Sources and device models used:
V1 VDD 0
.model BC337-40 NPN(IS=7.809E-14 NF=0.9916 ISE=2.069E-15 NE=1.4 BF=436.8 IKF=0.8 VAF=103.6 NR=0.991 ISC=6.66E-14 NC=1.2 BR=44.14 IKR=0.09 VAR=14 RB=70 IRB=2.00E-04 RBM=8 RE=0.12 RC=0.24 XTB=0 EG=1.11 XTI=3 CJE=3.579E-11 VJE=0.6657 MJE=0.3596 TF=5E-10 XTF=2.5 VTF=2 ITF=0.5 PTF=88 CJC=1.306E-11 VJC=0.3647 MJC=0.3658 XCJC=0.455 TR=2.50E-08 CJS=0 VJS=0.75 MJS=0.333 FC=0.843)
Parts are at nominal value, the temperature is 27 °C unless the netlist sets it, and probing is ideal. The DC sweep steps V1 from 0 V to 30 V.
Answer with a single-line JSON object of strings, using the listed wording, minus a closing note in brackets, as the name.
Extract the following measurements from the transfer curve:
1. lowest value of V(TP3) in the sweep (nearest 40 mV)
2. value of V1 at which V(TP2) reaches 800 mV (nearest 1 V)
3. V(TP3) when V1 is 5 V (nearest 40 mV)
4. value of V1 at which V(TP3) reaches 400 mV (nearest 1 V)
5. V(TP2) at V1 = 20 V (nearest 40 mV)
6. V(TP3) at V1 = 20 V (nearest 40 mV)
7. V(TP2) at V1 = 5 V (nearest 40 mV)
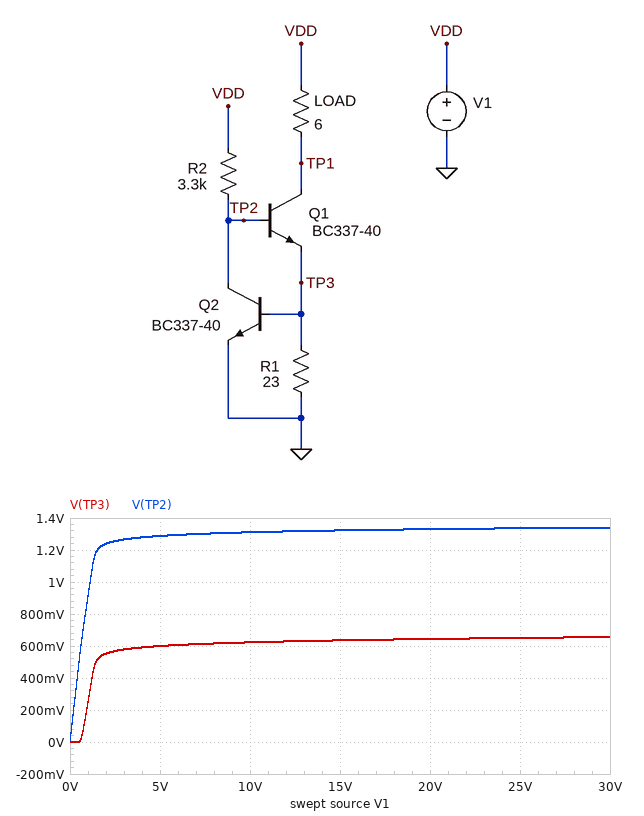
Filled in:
{"lowest value of V(TP3) in the sweep": "0 V", "value of V1 at which V(TP2) reaches 800 mV": "1 V", "V(TP3) when V1 is 5 V": "600 mV", "value of V1 at which V(TP3) reaches 400 mV": "1 V", "V(TP2) at V1 = 20 V": "1.32 V", "V(TP3) at V1 = 20 V": "640 mV", "V(TP2) at V1 = 5 V": "1.28 V"}
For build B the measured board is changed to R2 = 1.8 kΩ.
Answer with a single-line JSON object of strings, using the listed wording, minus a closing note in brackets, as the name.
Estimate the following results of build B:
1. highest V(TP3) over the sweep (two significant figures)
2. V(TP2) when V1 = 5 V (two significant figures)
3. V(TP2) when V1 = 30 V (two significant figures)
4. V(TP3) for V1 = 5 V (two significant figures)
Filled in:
{"highest V(TP3) over the sweep": "670 mV", "V(TP2) when V1 = 5 V": "1.3 V", "V(TP2) when V1 = 30 V": "1.4 V", "V(TP3) for V1 = 5 V": "620 mV"}
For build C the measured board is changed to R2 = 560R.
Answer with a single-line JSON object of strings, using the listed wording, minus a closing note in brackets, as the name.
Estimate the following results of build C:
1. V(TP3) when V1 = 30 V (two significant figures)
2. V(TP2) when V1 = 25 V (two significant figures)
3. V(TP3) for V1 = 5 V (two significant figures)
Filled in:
{"V(TP3) when V1 = 30 V": "710 mV", "V(TP2) when V1 = 25 V": "1.4 V", "V(TP3) for V1 = 5 V": "650 mV"}
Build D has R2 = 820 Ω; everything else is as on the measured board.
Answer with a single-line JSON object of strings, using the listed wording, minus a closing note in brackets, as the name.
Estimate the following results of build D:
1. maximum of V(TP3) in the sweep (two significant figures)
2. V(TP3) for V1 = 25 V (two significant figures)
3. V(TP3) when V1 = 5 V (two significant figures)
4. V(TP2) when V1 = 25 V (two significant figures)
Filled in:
{"maximum of V(TP3) in the sweep": "700 mV", "V(TP3) for V1 = 25 V": "690 mV", "V(TP3) when V1 = 5 V": "640 mV", "V(TP2) when V1 = 25 V": "1.4 V"}
